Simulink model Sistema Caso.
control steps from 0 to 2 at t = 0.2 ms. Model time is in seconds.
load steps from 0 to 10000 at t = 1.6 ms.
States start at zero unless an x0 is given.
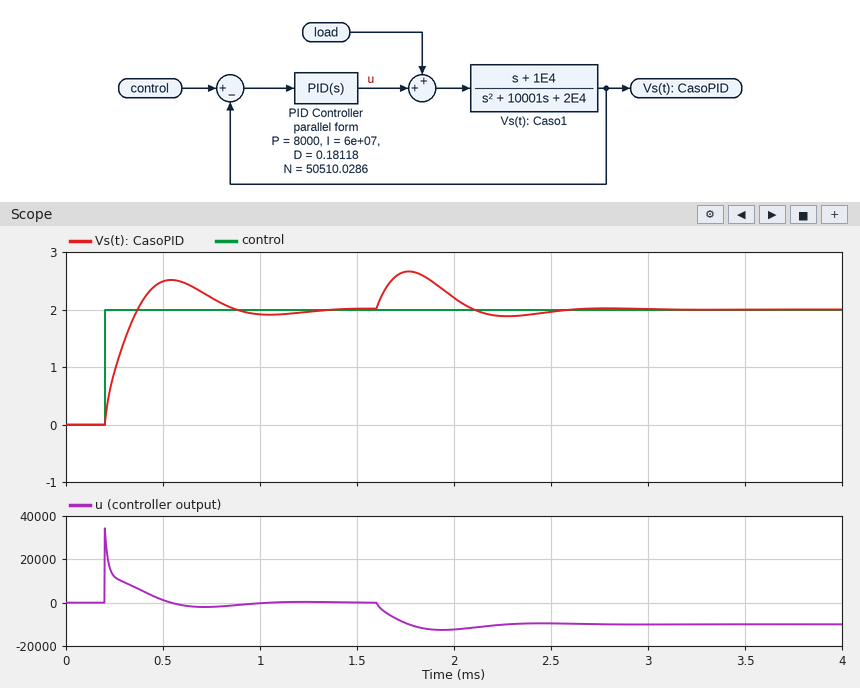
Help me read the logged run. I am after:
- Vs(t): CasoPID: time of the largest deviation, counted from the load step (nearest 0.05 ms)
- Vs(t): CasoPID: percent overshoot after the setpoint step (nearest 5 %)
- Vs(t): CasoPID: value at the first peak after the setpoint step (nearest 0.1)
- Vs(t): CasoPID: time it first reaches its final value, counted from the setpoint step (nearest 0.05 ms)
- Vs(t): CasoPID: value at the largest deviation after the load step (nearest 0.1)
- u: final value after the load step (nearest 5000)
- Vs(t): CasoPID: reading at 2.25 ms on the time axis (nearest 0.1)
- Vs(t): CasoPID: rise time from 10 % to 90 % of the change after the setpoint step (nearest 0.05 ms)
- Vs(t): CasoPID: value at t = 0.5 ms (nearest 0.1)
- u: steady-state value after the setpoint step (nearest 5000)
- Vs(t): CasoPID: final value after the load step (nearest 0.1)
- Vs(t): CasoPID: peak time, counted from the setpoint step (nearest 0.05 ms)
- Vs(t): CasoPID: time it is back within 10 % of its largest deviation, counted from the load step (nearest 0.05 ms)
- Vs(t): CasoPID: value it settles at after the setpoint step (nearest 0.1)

0.15 ms
25 %
2.5
0.15 ms
2.7
-10000
1.9
0.15 ms
2.5
0
2.0
0.35 ms
0.85 ms
2.0
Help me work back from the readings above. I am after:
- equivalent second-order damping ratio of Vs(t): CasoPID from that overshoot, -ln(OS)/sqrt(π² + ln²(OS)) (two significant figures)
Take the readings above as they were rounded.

0.40
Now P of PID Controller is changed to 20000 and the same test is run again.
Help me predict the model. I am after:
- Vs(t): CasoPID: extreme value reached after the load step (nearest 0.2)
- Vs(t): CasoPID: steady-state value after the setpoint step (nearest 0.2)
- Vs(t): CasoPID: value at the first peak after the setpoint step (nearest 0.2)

2.4
2.0
2.2
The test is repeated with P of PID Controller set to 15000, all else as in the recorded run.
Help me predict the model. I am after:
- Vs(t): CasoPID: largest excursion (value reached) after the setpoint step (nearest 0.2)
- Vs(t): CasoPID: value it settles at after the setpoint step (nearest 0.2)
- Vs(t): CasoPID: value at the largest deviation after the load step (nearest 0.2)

2.2
2.0
2.4
